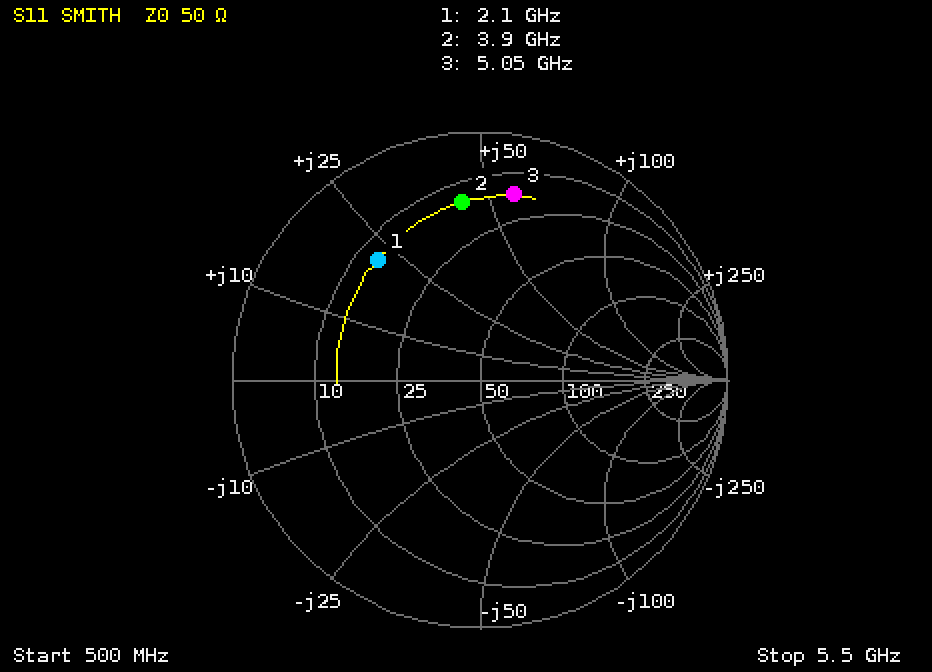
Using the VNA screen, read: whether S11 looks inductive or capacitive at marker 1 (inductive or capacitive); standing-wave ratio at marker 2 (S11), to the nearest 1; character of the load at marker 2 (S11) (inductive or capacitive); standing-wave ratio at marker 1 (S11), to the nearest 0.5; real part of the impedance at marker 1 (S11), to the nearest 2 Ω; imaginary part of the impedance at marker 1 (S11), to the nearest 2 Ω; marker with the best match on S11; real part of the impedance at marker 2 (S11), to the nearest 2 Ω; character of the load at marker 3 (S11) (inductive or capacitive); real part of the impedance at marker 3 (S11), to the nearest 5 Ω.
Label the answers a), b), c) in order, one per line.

a) inductive
b) 6
c) inductive
d) 4.5
e) 14 Ω
f) +22 Ω
g) marker 1
h) 14 Ω
i) inductive
j) 15 Ω
